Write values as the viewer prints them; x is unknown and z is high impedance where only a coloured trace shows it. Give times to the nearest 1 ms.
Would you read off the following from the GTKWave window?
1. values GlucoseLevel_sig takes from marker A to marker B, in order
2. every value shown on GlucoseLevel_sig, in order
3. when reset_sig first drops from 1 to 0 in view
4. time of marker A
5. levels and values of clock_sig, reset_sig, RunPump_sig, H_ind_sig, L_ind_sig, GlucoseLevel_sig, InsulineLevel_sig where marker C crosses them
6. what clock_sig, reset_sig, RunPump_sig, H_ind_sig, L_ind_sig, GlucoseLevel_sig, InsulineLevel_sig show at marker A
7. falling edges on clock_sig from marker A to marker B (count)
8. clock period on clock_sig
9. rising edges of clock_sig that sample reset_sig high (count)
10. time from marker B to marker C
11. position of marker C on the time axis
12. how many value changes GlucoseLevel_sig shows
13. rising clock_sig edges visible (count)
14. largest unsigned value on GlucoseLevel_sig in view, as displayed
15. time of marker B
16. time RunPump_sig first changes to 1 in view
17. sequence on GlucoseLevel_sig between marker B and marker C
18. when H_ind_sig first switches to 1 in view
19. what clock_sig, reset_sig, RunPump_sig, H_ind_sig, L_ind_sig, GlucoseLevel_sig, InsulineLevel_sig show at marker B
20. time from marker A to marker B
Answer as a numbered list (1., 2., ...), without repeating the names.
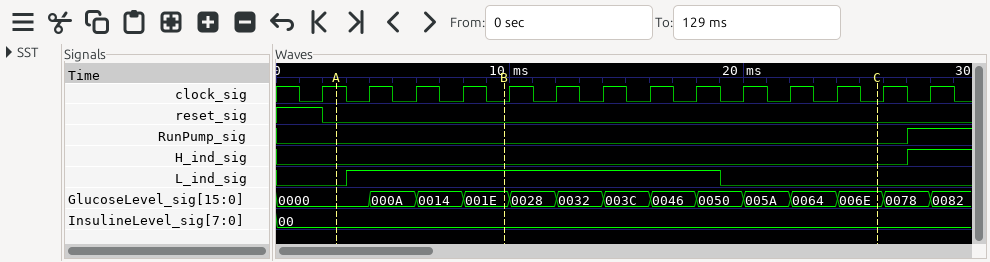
1. 0000, 000A, 0014, 001E
2. 0000, 000A, 0014, 001E, 0028, 0032, 003C, 0046, 0050, 005A, 0064, 006E, 0078, 0082
3. 2 ms
4. 3 ms
5. clock_sig=0, reset_sig=0, RunPump_sig=0, H_ind_sig=0, L_ind_sig=0, GlucoseLevel_sig=006E, InsulineLevel_sig=00
6. clock_sig=1, reset_sig=0, RunPump_sig=0, H_ind_sig=0, L_ind_sig=0, GlucoseLevel_sig=0000, InsulineLevel_sig=00
7. 4
8. 2 ms
9. 1
10. 16 ms
11. 26 ms
12. 13
13. 14
14. 0082
15. 10 ms
16. 27 ms
17. 001E, 0028, 0032, 003C, 0046, 0050, 005A, 0064, 006E
18. 27 ms
19. clock_sig=0, reset_sig=0, RunPump_sig=0, H_ind_sig=0, L_ind_sig=1, GlucoseLevel_sig=001E, InsulineLevel_sig=00
20. 7 ms
